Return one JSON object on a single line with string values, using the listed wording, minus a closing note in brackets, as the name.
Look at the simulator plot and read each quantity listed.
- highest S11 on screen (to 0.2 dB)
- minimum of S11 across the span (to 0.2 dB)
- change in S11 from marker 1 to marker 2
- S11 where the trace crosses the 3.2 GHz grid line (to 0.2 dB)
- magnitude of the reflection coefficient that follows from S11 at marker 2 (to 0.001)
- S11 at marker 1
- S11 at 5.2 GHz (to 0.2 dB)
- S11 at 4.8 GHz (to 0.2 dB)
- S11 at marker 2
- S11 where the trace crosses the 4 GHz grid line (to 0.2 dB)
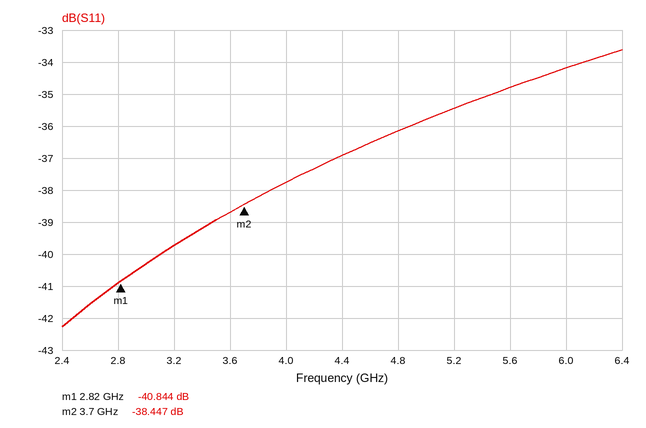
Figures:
{"highest S11 on screen": "-33.6 dB", "minimum of S11 across the span": "-42.2 dB", "change in S11 from marker 1 to marker 2": "2.397 dB", "S11 where the trace crosses the 3.2 GHz grid line": "-39.8 dB", "magnitude of the reflection coefficient that follows from S11 at marker 2": "0.012", "S11 at marker 1": "-40.844 dB", "S11 at 5.2 GHz": "-35.4 dB", "S11 at 4.8 GHz": "-36.2 dB", "S11 at marker 2": "-38.447 dB", "S11 where the trace crosses the 4 GHz grid line": "-37.8 dB"}
